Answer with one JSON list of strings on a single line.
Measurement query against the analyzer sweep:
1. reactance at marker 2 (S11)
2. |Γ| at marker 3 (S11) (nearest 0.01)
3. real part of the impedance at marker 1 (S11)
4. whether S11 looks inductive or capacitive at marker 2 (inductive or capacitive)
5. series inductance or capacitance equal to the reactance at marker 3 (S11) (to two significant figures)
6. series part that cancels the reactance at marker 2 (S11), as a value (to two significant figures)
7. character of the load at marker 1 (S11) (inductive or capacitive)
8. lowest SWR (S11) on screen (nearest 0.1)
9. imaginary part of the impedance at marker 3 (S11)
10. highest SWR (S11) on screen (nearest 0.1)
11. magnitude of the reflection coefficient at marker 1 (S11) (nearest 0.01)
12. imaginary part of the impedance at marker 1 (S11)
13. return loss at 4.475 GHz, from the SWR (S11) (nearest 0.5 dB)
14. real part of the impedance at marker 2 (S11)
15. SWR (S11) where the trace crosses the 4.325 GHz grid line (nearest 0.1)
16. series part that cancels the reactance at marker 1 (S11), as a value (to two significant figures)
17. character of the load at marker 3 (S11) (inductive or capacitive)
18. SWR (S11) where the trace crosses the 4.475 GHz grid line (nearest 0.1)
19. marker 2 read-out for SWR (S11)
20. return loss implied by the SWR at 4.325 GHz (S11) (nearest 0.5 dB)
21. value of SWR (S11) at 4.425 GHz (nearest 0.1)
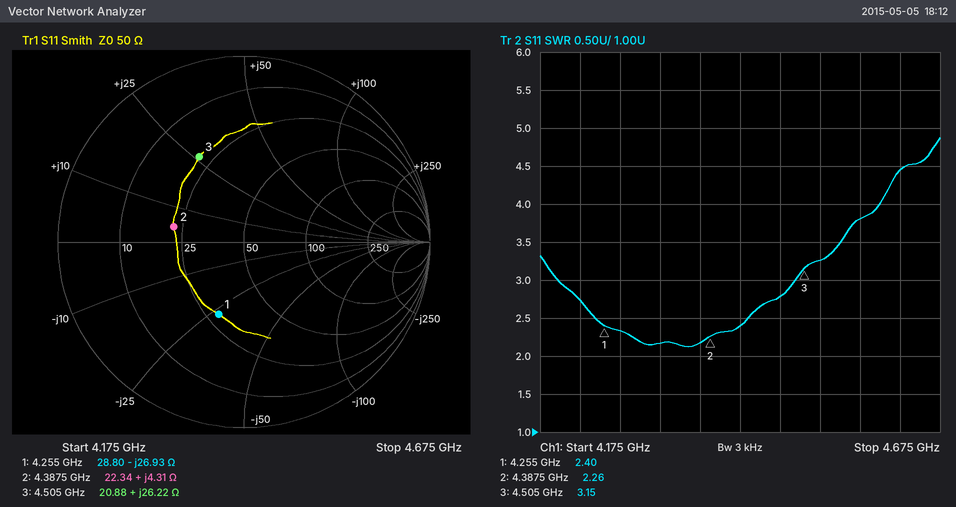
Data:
["+4.31 Ω", "0.52", "28.80 Ω", "inductive", "930 pH", "8.4 pF", "capacitive", "2.1", "+26.22 Ω", "4.9", "0.41", "-26.93 Ω", "6.5 dB", "22.34 Ω", "2.2", "1.0 nH", "inductive", "2.8", "2.26", "8.5 dB", "2.4"]
